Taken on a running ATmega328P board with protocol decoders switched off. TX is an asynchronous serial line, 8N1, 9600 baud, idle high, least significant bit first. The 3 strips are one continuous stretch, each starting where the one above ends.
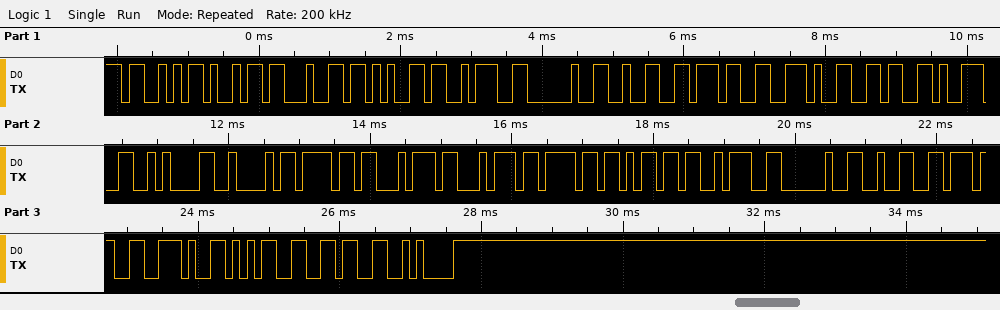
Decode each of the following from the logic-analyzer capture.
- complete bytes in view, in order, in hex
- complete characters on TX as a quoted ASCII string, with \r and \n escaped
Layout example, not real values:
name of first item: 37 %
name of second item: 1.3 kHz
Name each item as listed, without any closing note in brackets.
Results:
complete bytes in view, in order, in hex: 53 69 64 65 3A 20 32 37 2E 36 39 0A 42 6F 74 74 6F 6D 3A 20 32 37 2E 35 36 0A
complete characters on TX as a quoted ASCII string, with \r and \n escaped: "Side: 27.69\nBottom: 27.56\n"
